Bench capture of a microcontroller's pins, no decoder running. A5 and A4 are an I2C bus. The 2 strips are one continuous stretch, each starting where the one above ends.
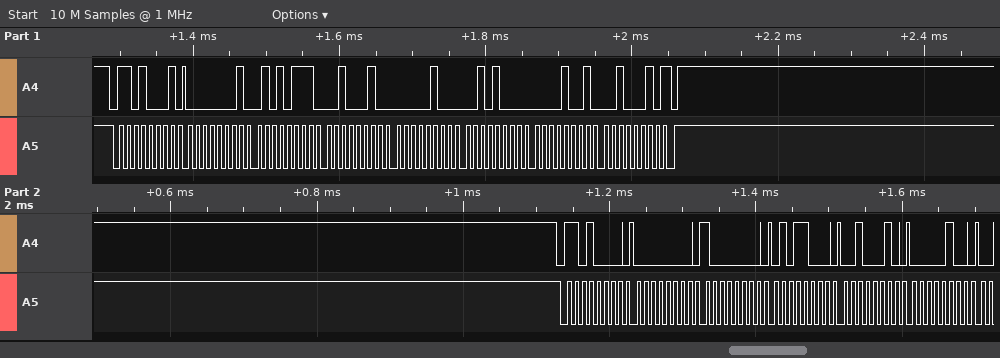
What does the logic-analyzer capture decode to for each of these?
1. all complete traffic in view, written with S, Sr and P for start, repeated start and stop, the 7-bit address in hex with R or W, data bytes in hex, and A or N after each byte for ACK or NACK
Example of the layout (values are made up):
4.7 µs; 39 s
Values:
S 68R A 01 A 57 A 22 A 04 A 28 A 09 A 22 N P S 68W A 00 A 80 A 58 A 22 A 04 A
